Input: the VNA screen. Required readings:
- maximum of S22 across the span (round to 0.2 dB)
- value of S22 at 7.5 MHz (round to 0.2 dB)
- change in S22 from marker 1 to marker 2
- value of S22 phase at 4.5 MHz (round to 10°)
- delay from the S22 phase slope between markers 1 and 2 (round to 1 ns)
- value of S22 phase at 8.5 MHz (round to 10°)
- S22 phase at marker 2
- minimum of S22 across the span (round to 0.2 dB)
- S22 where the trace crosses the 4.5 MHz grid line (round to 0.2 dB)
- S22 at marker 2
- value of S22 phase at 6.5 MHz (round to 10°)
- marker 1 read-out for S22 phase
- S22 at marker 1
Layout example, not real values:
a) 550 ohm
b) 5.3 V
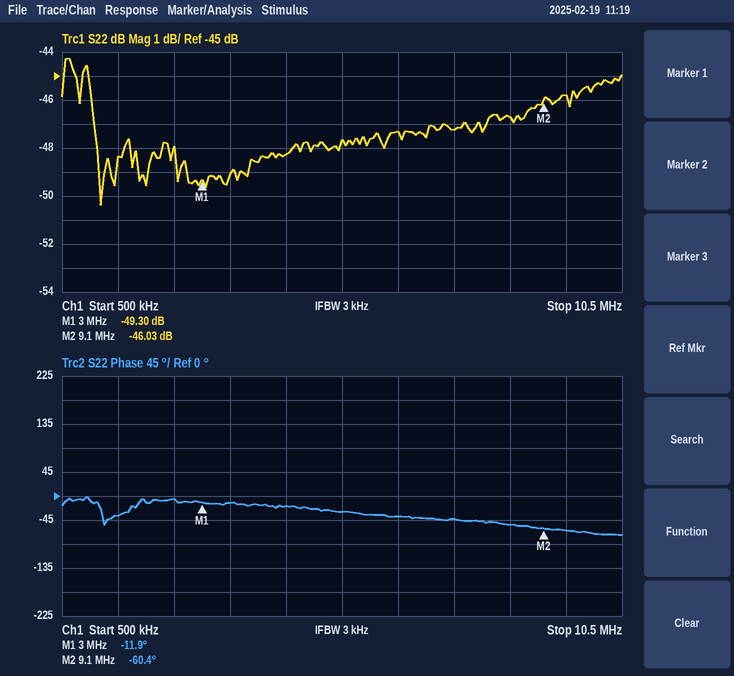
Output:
a) -44.2 dB
b) -47.2 dB
c) 3.27 dB
d) -20°
e) 22 ns
f) -50°
g) -60.4°
h) -50.4 dB
i) -48.2 dB
j) -46.03 dB
k) -40°
l) -11.9°
m) -49.30 dB
